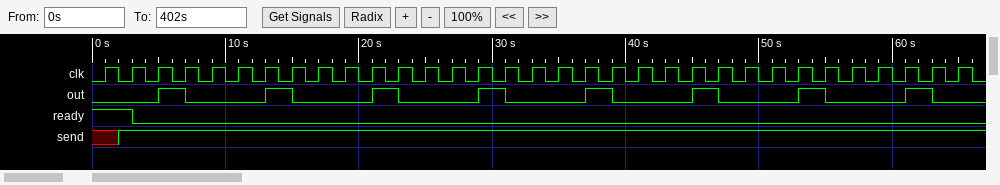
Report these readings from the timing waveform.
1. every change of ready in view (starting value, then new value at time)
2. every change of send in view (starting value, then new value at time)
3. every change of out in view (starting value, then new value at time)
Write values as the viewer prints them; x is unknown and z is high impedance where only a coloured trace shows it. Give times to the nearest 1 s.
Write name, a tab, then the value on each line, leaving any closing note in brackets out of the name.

every change of ready in view	1, 0 at 3 s
every change of send in view	x, 1 at 2 s
every change of out in view	0, 1 at 5 s, 0 at 7 s, 1 at 13 s, 0 at 15 s, 1 at 21 s, 0 at 23 s, 1 at 29 s, 0 at 31 s, 1 at 37 s, 0 at 39 s, 1 at 45 s, 0 at 47 s, 1 at 53 s, 0 at 55 s, 1 at 61 s, 0 at 63 s
